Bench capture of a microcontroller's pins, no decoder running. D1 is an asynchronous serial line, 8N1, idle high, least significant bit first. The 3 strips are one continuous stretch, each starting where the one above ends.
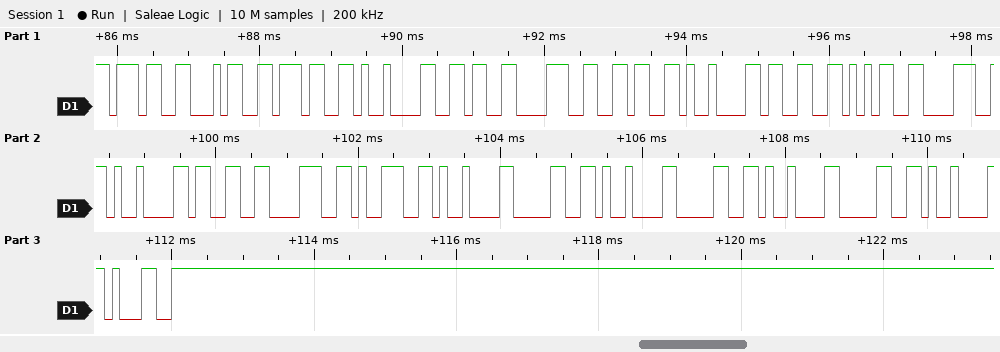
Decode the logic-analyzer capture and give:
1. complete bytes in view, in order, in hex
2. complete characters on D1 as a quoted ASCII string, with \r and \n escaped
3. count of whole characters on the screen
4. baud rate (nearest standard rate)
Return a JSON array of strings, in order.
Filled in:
["0x37 0x34 0x37 0x09 0x36 0x38 0x36 0x09 0x33 0x35 0x38 0x09 0x33 0x38 0x39 0x09 0x30 0x09 0x30 0x09 0x30 0x09 0x31", "\"747\\t686\\t358\\t389\\t0\\t0\\t0\\t1\"", "23", "9600 baud"]
